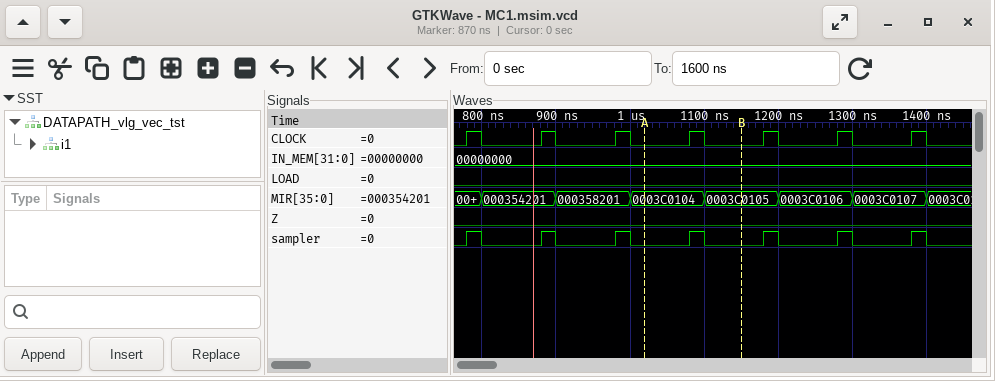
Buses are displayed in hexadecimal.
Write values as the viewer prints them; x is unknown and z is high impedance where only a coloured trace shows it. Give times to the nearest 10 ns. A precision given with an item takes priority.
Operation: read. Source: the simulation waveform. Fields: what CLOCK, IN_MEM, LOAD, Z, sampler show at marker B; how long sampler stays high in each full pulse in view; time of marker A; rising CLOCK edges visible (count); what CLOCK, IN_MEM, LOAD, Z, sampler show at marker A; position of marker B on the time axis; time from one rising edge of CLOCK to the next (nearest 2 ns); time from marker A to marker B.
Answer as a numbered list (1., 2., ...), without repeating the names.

1. CLOCK=0, IN_MEM=00000000, LOAD=0, Z=0, sampler=0
2. 20 ns, 20 ns, 20 ns, 20 ns, 20 ns, 20 ns, 20 ns
3. 1020 ns
4. 7
5. CLOCK=0, IN_MEM=00000000, LOAD=0, Z=0, sampler=0
6. 1150 ns
7. 100 ns
8. 130 ns
